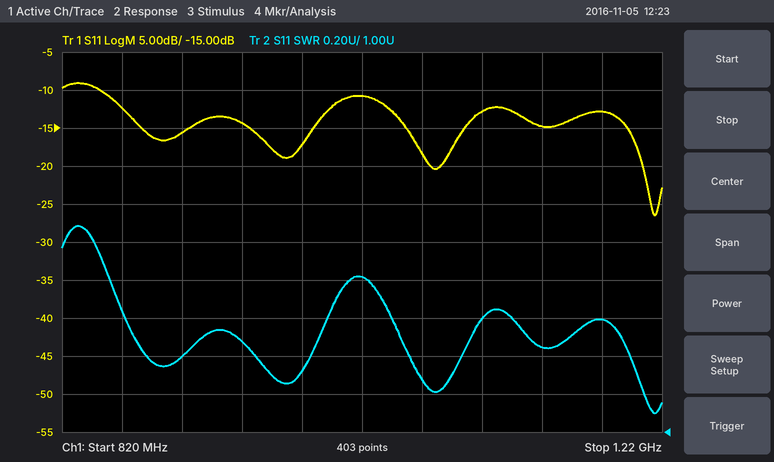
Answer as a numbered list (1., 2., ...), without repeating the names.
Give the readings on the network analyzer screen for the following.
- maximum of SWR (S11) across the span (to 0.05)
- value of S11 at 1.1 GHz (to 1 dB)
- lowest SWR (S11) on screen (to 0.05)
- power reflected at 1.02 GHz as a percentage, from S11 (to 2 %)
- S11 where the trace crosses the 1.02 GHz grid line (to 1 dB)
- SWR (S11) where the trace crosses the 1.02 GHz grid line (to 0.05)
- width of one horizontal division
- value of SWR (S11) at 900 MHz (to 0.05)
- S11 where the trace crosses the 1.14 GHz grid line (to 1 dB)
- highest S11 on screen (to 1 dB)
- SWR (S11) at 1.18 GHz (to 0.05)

1. 2.10
2. -13 dB
3. 1.10
4. 8 %
5. -11 dB
6. 1.80
7. 40 MHz
8. 1.40
9. -15 dB
10. -9 dB
11. 1.60
